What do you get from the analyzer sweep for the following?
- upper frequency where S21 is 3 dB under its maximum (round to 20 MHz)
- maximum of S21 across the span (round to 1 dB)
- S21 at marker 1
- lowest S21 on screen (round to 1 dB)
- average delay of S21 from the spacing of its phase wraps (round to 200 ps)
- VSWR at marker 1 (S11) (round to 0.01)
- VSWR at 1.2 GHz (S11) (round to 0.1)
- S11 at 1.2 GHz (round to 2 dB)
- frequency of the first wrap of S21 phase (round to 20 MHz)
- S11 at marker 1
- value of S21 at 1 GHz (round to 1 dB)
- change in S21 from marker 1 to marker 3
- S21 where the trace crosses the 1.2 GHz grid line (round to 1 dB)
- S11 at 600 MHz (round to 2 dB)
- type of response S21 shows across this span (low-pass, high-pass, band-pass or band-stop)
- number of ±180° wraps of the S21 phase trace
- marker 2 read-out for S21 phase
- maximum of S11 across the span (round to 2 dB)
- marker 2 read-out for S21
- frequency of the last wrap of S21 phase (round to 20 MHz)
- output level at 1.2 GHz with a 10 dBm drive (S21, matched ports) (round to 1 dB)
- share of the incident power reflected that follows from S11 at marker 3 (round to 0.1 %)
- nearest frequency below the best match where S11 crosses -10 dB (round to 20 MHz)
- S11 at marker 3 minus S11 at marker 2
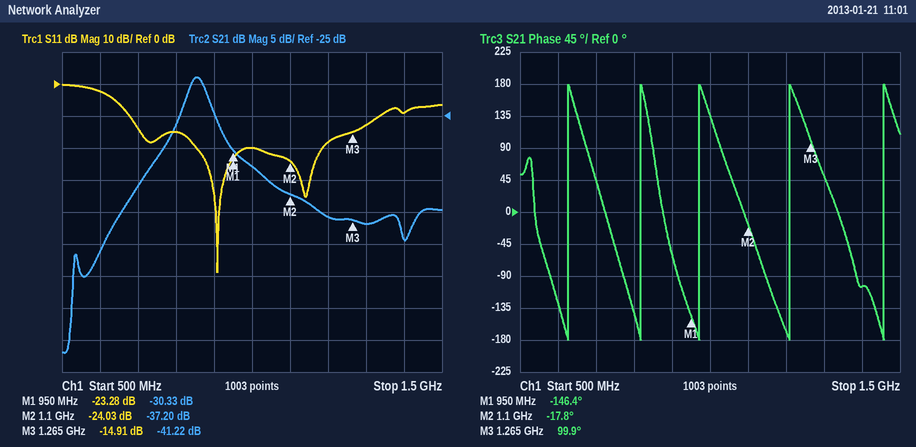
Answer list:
880 MHz
-19 dB
-30.33 dB
-62 dB
4.8 ns
1.15
1.3
-18 dB
620 MHz
-23.28 dB
-33 dB
-10.89 dB
-41 dB
-2 dB
band-pass
5
-17.8°
0 dB
-37.20 dB
1.46 GHz
-31 dBm
3.2 %
680 MHz
9.12 dB
